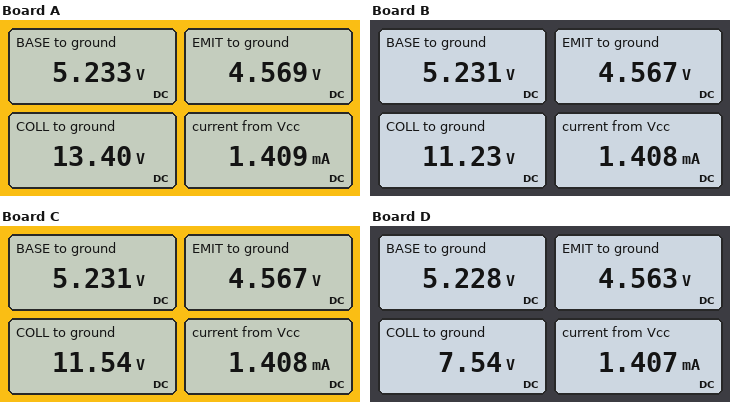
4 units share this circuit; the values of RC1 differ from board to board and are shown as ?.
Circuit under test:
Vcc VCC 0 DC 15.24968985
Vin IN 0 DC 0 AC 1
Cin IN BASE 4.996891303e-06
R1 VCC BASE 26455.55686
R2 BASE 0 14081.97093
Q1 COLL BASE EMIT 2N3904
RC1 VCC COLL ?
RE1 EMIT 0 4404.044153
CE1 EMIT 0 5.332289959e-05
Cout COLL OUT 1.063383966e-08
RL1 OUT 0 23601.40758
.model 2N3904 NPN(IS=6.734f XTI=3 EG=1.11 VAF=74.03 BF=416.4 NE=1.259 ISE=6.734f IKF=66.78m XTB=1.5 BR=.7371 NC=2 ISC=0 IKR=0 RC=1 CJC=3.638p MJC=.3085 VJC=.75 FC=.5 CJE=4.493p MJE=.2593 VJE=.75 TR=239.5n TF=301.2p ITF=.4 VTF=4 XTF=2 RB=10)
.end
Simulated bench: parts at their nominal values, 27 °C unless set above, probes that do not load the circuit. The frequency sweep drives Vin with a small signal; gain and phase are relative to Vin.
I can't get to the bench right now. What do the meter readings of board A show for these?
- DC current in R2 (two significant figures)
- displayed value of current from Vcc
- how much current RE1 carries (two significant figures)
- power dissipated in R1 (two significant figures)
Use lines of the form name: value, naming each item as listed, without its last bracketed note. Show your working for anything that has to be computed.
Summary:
DC current in R2: (5.233 V) / 14.08 kΩ = 370 µA
displayed value of current from Vcc: 1.409 mA
how much current RE1 carries: (4.569 V) / 4.404 kΩ = 1.0 mA
power dissipated in R1: (15.25 V - 5.233 V)^2 / 26.46 kΩ = 3.8 mW
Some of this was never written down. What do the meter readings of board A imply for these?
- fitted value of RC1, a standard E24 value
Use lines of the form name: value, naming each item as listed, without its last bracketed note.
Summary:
fitted value of RC1, a standard E24 value: 1.8 kΩ
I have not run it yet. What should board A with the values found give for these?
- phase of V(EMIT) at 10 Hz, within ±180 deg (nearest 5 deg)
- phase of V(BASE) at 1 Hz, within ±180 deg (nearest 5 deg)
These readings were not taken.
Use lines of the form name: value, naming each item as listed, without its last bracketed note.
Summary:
phase of V(EMIT) at 10 Hz, within ±180 deg: 15 deg
phase of V(BASE) at 1 Hz, within ±180 deg: 75 deg
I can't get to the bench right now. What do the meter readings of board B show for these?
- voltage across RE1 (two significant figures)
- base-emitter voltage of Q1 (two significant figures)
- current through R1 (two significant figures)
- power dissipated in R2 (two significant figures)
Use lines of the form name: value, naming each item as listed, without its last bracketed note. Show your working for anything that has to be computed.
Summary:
voltage across RE1: 4.567 V = 4.6 V
base-emitter voltage of Q1: 5.231 V - 4.567 V = 660 mV
current through R1: (15.25 V - 5.231 V) / 26.46 kΩ = 380 µA
power dissipated in R2: (5.231 V)^2 / 14.08 kΩ = 1.9 mW
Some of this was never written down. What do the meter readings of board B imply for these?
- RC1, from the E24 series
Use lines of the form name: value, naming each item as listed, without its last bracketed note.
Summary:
RC1, from the E24 series: 3.9 kΩ
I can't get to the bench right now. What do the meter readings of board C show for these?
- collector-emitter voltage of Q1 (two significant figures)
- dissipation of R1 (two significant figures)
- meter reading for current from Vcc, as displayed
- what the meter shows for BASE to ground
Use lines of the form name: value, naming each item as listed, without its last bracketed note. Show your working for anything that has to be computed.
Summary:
collector-emitter voltage of Q1: 11.54 V - 4.567 V = 7.0 V
dissipation of R1: (15.25 V - 5.231 V)^2 / 26.46 kΩ = 3.8 mW
meter reading for current from Vcc, as displayed: 1.408 mA
what the meter shows for BASE to ground: 5.231 V
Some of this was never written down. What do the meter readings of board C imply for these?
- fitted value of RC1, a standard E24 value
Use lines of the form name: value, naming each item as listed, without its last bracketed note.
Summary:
fitted value of RC1, a standard E24 value: 3.6 kΩ
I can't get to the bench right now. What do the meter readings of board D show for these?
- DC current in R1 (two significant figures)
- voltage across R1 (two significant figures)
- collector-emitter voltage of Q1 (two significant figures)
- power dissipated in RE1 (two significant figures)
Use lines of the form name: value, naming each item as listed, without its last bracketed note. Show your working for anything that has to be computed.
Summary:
DC current in R1: (15.25 V - 5.228 V) / 26.46 kΩ = 380 µA
voltage across R1: 15.25 V - 5.228 V = 10 V
collector-emitter voltage of Q1: 7.54 V - 4.563 V = 3.0 V
power dissipated in RE1: (4.563 V)^2 / 4.404 kΩ = 4.7 mW
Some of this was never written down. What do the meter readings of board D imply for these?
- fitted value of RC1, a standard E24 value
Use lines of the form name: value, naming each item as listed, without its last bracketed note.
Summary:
fitted value of RC1, a standard E24 value: 7.5 kΩ
